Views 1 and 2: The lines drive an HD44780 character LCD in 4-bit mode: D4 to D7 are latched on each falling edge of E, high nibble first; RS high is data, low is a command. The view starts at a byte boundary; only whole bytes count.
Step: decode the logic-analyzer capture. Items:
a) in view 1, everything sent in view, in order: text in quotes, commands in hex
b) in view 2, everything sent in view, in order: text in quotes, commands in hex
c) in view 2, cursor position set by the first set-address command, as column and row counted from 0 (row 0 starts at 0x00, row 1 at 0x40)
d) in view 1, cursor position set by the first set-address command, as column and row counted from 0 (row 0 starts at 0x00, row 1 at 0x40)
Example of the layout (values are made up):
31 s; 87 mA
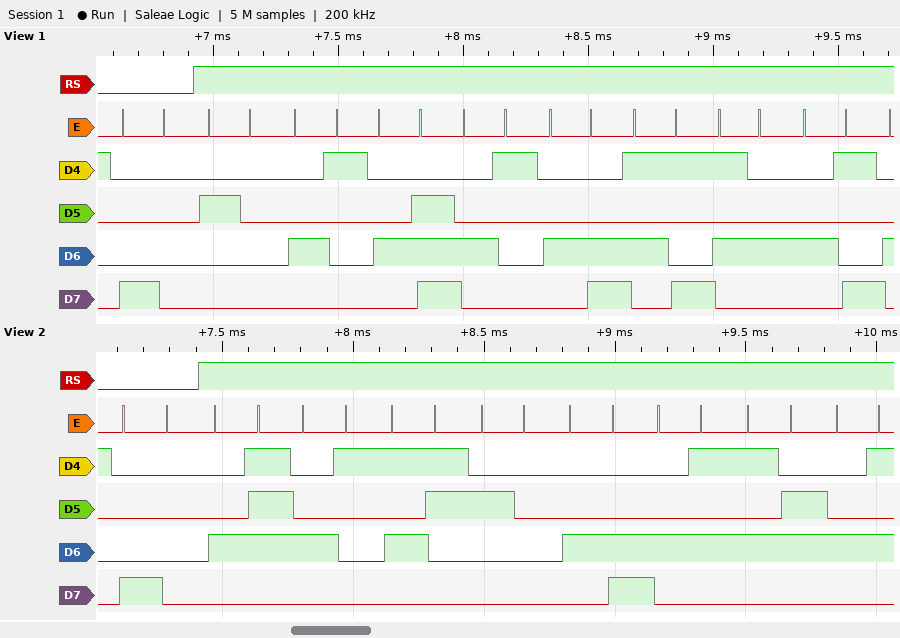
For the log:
0x80 " ANALYTI"; 0x80 "GAS LEVE"; column 0, row 0; column 0, row 0
